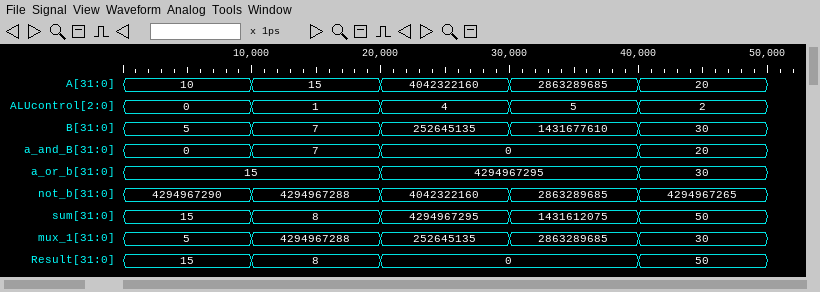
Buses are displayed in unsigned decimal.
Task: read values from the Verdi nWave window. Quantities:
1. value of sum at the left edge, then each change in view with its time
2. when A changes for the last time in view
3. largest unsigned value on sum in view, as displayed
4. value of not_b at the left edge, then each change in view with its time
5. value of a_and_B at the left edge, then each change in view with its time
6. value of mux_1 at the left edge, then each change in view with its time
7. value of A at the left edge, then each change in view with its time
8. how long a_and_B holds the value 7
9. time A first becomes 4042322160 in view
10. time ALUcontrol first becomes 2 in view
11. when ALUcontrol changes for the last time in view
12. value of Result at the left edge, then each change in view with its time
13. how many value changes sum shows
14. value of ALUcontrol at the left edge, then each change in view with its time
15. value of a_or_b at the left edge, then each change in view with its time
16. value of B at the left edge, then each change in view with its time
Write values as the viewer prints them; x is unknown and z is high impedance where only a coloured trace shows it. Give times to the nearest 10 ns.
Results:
15, 8 at 10 ns, 4294967295 at 20 ns, 1431612075 at 30 ns, 50 at 40 ns
40 ns
4294967295
4294967290, 4294967288 at 10 ns, 4042322160 at 20 ns, 2863289685 at 30 ns, 4294967265 at 40 ns
0, 7 at 10 ns, 0 at 20 ns, 20 at 40 ns
5, 4294967288 at 10 ns, 252645135 at 20 ns, 2863289685 at 30 ns, 30 at 40 ns
10, 15 at 10 ns, 4042322160 at 20 ns, 2863289685 at 30 ns, 20 at 40 ns
10 ns
20 ns
40 ns
40 ns
15, 8 at 10 ns, 0 at 20 ns, 50 at 40 ns
4
0, 1 at 10 ns, 4 at 20 ns, 5 at 30 ns, 2 at 40 ns
15, 4294967295 at 20 ns, 30 at 40 ns
5, 7 at 10 ns, 252645135 at 20 ns, 1431677610 at 30 ns, 30 at 40 ns
